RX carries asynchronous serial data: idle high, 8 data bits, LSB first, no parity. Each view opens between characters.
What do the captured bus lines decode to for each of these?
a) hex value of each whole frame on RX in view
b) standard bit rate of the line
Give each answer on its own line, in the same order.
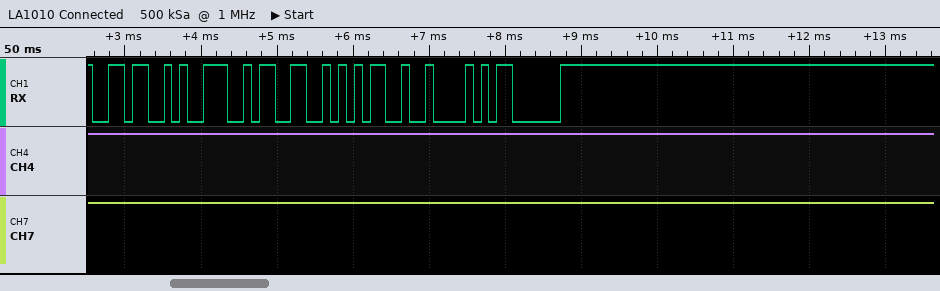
36, 39, 33, 35, 42, 03
9600 baud
